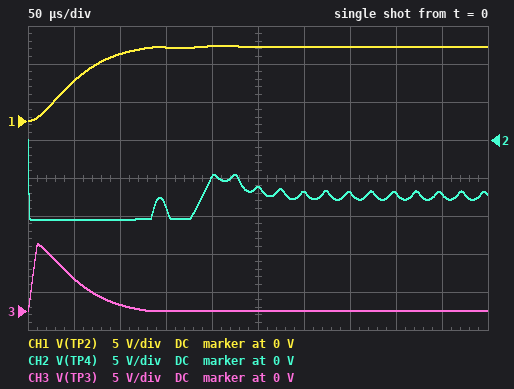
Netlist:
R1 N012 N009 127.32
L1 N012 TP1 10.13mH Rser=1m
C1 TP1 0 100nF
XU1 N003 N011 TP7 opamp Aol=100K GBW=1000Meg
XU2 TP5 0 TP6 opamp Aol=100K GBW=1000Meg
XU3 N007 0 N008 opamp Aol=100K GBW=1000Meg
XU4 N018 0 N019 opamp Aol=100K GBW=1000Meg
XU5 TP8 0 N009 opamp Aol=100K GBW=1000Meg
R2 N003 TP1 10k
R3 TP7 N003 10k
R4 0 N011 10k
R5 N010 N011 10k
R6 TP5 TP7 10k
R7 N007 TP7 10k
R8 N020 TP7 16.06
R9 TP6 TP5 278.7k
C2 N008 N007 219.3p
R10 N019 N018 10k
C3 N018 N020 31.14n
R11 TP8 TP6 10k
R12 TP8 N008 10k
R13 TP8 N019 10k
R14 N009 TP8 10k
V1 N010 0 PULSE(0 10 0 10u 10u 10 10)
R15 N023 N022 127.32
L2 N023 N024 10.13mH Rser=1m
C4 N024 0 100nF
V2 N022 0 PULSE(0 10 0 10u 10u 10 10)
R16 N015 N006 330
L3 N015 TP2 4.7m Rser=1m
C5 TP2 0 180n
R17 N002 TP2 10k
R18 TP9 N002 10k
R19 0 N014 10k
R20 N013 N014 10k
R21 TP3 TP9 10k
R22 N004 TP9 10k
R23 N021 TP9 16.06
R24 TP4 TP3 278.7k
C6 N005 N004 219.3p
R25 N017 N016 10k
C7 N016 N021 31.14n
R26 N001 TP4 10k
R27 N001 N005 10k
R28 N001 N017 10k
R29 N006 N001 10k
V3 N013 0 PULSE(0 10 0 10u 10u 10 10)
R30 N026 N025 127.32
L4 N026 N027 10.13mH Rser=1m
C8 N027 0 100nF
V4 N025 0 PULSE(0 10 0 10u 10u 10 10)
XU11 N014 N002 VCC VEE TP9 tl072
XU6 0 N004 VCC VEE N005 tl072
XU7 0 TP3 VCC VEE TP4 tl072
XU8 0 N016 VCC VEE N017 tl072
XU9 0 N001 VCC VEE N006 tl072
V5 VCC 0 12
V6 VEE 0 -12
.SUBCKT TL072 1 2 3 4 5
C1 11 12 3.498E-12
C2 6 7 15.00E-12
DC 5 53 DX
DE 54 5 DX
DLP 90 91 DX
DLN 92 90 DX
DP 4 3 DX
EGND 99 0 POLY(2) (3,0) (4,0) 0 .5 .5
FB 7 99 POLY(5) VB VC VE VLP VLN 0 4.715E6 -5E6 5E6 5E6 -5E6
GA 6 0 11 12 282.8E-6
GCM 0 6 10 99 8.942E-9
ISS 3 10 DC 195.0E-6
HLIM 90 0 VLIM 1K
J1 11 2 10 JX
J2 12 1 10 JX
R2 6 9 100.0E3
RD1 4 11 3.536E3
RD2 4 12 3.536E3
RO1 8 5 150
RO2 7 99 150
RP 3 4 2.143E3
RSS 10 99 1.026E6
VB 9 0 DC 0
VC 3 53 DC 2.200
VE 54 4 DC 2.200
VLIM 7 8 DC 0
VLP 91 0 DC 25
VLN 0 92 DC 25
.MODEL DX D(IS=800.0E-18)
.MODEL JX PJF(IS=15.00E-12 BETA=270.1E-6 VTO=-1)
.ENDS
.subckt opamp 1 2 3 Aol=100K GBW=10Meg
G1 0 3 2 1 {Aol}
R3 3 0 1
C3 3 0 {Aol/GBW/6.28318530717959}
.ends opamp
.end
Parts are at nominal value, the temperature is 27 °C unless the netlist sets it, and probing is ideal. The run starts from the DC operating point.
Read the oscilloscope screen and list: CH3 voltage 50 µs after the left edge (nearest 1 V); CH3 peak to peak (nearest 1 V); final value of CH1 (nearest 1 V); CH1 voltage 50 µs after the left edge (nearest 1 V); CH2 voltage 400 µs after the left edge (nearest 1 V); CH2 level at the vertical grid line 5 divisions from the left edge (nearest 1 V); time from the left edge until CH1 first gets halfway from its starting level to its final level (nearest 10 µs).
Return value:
4 V
9 V
10 V
5 V
-7 V
-6 V
50 µs
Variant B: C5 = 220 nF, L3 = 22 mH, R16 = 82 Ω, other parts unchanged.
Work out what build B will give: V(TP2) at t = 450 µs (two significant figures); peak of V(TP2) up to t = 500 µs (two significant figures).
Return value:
7.2 V
11 V
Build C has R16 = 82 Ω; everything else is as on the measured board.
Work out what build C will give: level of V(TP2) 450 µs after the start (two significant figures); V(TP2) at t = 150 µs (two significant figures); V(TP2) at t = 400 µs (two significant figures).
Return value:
9.9 V
7.5 V
8.7 V
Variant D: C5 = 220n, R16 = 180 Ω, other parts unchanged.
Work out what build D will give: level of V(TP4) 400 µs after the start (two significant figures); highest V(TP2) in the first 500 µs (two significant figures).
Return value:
-7.3 V
10 V
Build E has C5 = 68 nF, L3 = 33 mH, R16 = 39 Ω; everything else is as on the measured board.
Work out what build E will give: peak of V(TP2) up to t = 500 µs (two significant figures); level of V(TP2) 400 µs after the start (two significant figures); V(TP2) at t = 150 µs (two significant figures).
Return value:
14 V
-2.1 V
2.8 V
